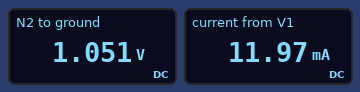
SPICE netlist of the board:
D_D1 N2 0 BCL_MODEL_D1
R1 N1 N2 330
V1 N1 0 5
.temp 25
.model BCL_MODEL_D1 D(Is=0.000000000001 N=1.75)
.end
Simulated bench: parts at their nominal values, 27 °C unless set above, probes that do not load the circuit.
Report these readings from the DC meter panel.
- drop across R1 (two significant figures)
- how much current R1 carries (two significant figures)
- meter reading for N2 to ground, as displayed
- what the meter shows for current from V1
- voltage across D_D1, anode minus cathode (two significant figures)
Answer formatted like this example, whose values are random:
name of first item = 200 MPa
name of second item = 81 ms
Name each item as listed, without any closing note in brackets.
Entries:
drop across R1 = 3.9 V
how much current R1 carries = 12 mA
meter reading for N2 to ground, as displayed = 1.051 V
what the meter shows for current from V1 = 11.97 mA
voltage across D_D1, anode minus cathode = 1.1 V
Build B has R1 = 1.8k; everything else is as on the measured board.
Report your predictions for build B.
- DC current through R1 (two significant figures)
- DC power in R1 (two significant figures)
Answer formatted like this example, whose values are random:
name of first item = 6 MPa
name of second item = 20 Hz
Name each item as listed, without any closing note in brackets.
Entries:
DC current through R1 = 2.2 mA
DC power in R1 = 9.0 mW
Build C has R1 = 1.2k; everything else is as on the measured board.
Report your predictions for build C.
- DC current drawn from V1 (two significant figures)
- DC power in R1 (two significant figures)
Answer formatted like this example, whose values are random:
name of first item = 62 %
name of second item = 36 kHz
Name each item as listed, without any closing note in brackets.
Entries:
DC current drawn from V1 = 3.3 mA
DC power in R1 = 13 mW
